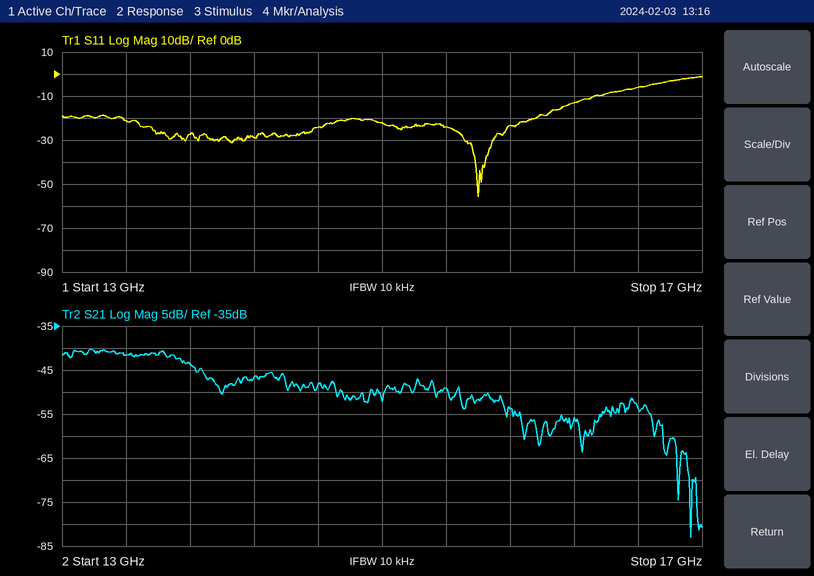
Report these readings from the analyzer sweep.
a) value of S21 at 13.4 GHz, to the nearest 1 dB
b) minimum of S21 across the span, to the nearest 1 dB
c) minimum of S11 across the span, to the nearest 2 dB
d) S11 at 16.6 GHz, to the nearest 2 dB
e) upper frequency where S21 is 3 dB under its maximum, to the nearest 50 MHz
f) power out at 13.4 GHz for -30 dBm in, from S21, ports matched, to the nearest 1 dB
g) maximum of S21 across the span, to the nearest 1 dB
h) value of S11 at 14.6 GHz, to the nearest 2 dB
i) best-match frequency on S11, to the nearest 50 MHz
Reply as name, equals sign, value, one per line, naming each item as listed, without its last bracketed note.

value of S21 at 13.4 GHz, to the nearest 1 dB = -42 dB
minimum of S21 across the span, to the nearest 1 dB = -83 dB
minimum of S11 across the span, to the nearest 2 dB = -56 dB
S11 at 16.6 GHz, to the nearest 2 dB = -6 dB
upper frequency where S21 is 3 dB under its maximum, to the nearest 50 MHz = 13.75 GHz
power out at 13.4 GHz for -30 dBm in, from S21, ports matched, to the nearest 1 dB = -72 dBm
maximum of S21 across the span, to the nearest 1 dB = -40 dB
value of S11 at 14.6 GHz, to the nearest 2 dB = -24 dB
best-match frequency on S11, to the nearest 50 MHz = 15.60 GHz
